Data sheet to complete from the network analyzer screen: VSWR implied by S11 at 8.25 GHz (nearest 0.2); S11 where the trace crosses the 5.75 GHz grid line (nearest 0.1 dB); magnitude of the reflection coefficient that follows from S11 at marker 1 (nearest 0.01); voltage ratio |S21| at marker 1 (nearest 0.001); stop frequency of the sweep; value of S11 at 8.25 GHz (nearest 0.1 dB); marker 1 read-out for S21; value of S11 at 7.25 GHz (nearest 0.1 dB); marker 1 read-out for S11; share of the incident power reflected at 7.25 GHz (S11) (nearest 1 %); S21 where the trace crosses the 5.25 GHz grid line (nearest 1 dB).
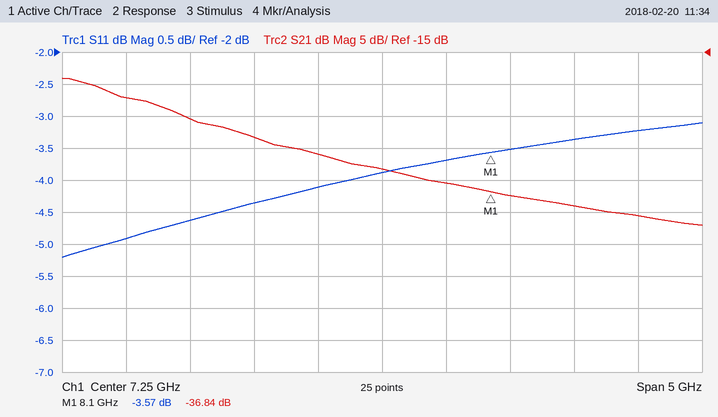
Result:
5.0
-4.6 dB
0.66
0.014
9.75 GHz
-3.5 dB
-36.84 dB
-3.9 dB
-3.57 dB
41 %
-22 dB
